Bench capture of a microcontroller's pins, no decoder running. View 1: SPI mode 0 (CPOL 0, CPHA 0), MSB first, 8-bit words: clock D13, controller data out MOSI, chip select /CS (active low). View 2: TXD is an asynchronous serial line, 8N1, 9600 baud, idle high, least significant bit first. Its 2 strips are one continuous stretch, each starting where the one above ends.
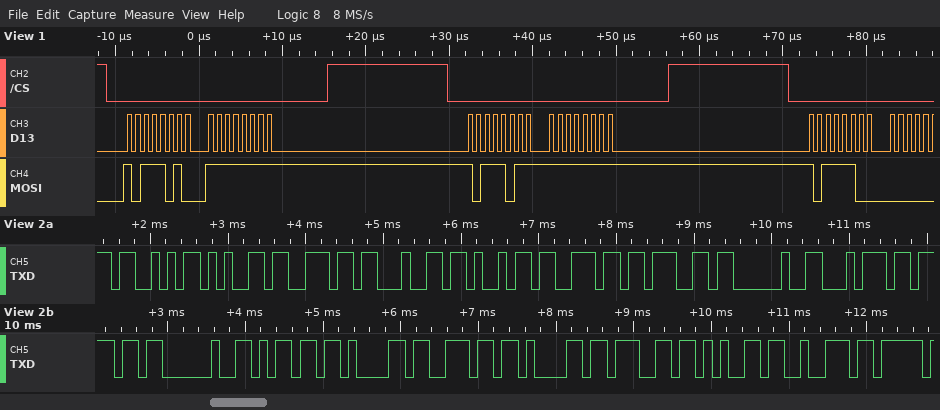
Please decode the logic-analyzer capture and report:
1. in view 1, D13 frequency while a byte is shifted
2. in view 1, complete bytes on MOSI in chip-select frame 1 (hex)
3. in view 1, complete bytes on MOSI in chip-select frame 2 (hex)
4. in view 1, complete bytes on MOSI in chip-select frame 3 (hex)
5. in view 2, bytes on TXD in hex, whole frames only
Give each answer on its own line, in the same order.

1 MHz
BA FF
BB FF
BC
53 65 6E 64 69 6E 67 20 74 6F 20 6D 61 6E 61 67 65 72
